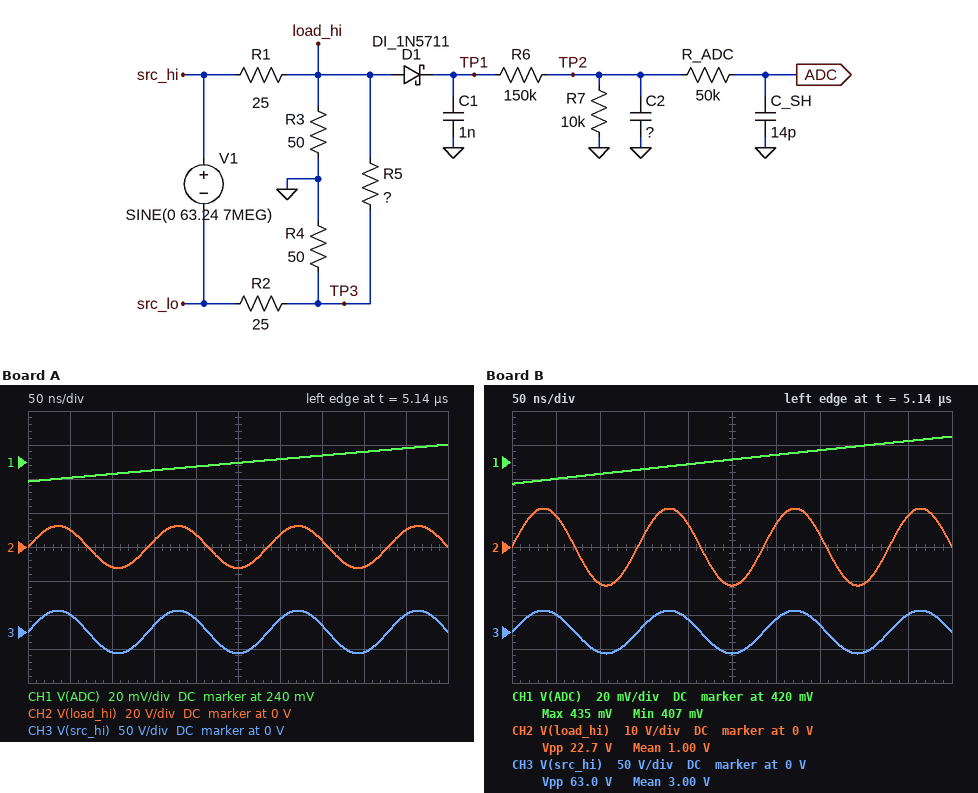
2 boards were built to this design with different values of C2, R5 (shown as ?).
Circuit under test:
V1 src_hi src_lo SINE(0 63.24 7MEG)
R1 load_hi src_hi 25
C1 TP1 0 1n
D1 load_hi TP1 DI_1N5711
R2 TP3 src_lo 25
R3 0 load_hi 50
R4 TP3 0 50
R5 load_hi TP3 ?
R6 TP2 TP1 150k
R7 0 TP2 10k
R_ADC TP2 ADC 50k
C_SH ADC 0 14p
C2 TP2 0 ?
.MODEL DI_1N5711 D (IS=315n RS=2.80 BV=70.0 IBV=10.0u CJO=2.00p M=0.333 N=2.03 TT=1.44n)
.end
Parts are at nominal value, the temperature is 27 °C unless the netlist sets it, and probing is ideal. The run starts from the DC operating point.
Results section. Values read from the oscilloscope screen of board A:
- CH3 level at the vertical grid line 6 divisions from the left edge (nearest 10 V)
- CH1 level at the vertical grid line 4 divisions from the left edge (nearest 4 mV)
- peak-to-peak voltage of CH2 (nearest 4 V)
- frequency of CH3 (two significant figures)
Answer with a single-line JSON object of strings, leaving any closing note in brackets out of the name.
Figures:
{"CH3 level at the vertical grid line 6 divisions from the left edge": "20 V", "CH1 level at the vertical grid line 4 divisions from the left edge": "236 mV", "peak-to-peak voltage of CH2": "24 V", "frequency of CH3": "7.0 MHz"}
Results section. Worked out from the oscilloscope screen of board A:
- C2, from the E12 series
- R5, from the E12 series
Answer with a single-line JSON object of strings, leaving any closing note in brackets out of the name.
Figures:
{"C2, from the E12 series": "1.2 nF", "R5, from the E12 series": "47 Ω"}
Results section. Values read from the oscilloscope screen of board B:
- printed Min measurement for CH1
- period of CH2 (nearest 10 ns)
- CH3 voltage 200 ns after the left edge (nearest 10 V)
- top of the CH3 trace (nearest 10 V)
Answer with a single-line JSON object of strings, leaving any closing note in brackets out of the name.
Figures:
{"printed Min measurement for CH1": "407 mV", "period of CH2": "140 ns", "CH3 voltage 200 ns after the left edge": "20 V", "top of the CH3 trace": "30 V"}
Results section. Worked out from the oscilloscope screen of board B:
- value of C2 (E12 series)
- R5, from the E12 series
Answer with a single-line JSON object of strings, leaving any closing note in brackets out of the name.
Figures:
{"value of C2": "470 pF", "R5, from the E12 series": "39 Ω"}
